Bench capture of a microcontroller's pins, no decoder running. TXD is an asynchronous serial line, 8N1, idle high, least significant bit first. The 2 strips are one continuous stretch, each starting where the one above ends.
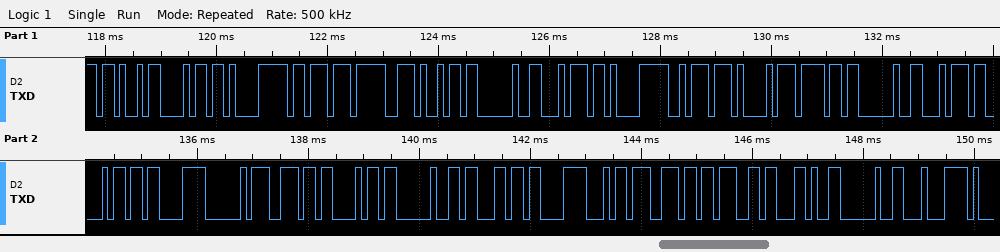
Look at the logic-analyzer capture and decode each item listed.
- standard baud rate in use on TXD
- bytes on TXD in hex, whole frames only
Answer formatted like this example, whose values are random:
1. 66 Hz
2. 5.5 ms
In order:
1. 9600 baud
2. 0x4B 0x68 0xE1 0xBB 0x9F 0x69 0x20 0x74 0xE1 0xBA 0xA1 0x6F 0x20 0x74 0x68 0xC3 0xA0 0x6E 0x68 0x20 0x63 0xC3 0xB4 0x6E 0x67 0x2C 0x20 0xC4
